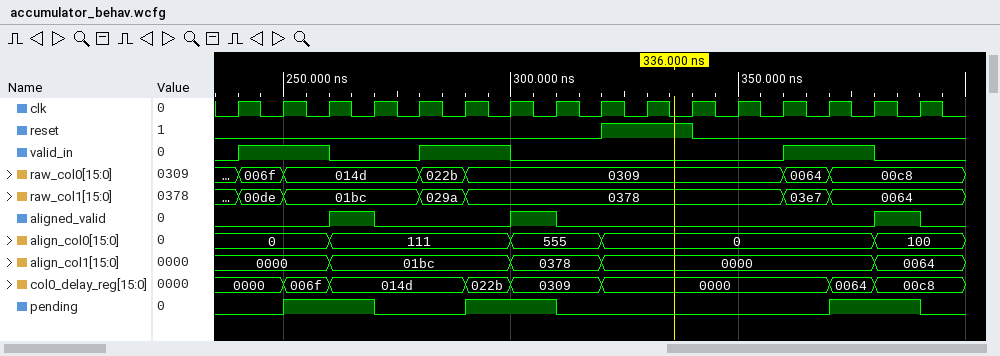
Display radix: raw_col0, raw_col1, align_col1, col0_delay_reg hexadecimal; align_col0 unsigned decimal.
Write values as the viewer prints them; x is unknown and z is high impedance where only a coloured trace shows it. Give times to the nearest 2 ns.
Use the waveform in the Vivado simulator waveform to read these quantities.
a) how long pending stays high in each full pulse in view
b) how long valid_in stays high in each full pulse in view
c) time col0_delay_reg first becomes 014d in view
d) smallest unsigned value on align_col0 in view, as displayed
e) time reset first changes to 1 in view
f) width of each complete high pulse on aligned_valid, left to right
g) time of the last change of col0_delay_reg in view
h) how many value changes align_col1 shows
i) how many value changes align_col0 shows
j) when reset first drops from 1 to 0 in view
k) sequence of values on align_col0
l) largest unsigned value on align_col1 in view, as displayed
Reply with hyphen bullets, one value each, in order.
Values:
- 20 ns, 20 ns, 20 ns
- 20 ns, 20 ns, 20 ns
- 260 ns
- 0
- 320 ns
- 10 ns, 10 ns, 10 ns
- 380 ns
- 4
- 4
- 340 ns
- 0, 111, 555, 0, 100
- 0378
